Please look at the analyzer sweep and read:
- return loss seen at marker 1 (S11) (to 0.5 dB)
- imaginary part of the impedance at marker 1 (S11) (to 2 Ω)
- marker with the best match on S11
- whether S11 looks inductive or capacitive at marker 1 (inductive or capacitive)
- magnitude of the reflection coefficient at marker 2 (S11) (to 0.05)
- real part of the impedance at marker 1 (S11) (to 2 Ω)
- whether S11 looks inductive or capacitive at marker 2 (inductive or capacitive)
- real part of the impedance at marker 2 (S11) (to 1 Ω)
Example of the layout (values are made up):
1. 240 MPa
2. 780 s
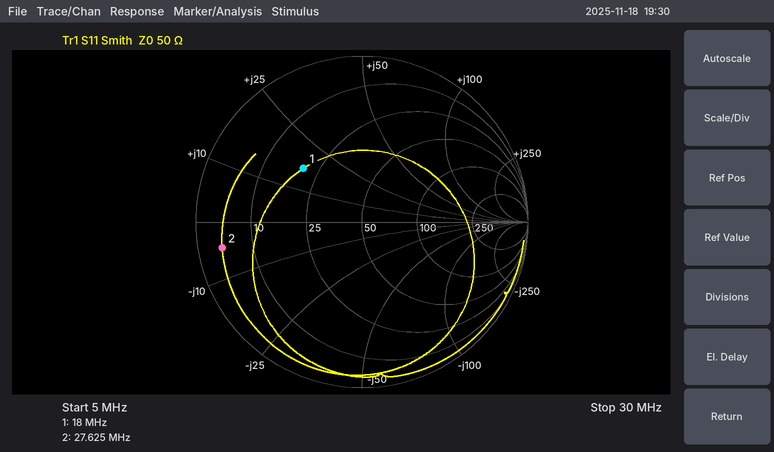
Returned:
1. 6.5 dB
2. +16 Ω
3. marker 1
4. inductive
5. 0.85
6. 20 Ω
7. capacitive
8. 4 Ω
